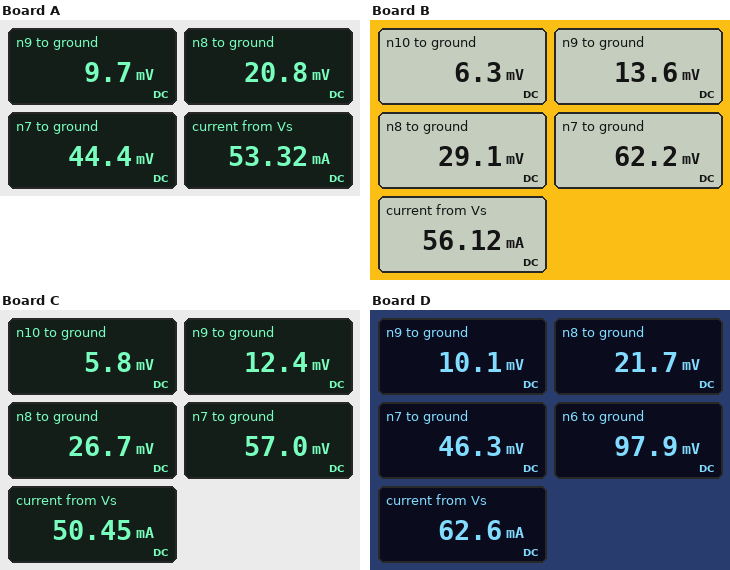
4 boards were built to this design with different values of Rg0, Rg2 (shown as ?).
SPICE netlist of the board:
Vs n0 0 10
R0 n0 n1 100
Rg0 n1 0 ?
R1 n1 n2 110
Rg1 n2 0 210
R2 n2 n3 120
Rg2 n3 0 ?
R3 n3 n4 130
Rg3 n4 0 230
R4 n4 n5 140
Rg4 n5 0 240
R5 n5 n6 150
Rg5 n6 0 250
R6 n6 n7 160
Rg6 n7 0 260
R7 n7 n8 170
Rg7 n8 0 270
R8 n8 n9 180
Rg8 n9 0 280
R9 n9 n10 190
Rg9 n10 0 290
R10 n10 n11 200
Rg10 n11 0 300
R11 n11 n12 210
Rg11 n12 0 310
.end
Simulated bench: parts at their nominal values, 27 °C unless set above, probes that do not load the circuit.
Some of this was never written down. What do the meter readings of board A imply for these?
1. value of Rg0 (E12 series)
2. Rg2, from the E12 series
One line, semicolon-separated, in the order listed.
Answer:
150 Ω; 100 Ω
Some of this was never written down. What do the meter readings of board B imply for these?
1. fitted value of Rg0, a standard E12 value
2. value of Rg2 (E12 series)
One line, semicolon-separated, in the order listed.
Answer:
120 Ω; 270 Ω
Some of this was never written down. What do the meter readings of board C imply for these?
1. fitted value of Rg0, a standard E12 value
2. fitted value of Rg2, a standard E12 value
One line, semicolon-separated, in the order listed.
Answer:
180 Ω; 150 Ω
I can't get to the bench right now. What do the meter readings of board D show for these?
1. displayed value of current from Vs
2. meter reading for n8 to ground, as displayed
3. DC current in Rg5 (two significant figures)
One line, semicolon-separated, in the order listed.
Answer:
62.6 mA; 21.7 mV; 390 µA
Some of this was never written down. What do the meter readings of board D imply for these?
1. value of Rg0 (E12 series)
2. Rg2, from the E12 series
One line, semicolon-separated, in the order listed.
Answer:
82 Ω; 180 Ω
